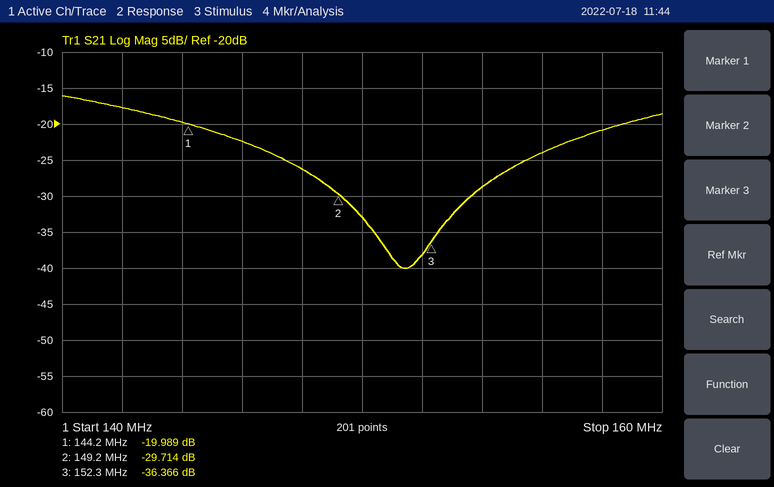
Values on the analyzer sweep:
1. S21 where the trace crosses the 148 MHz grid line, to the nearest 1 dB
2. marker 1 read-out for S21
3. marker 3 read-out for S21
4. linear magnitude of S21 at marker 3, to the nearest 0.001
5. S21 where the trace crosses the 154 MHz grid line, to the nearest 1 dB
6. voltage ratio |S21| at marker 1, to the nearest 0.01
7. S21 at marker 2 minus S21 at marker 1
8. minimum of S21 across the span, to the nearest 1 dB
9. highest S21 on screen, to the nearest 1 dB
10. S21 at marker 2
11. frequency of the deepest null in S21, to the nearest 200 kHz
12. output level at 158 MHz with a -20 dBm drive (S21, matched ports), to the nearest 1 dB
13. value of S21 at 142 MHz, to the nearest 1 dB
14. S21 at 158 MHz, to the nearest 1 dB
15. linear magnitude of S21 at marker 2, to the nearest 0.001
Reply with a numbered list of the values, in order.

1. -26 dB
2. -19.989 dB
3. -36.366 dB
4. 0.015
5. -29 dB
6. 0.10
7. -9.725 dB
8. -40 dB
9. -16 dB
10. -29.714 dB
11. 151.4 MHz
12. -41 dBm
13. -18 dB
14. -21 dB
15. 0.033
